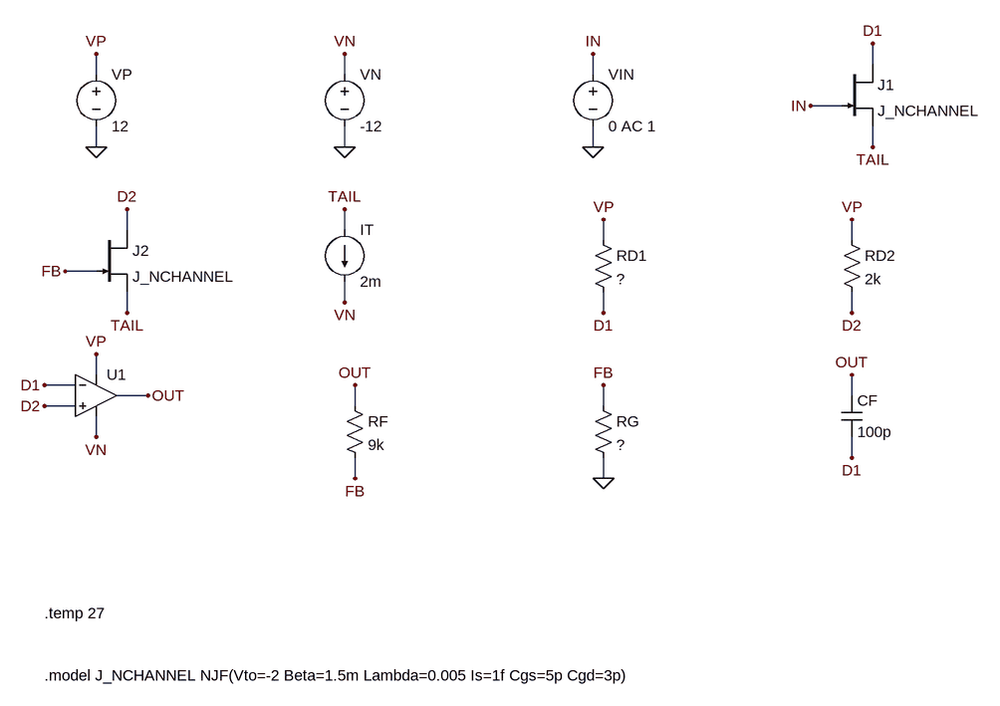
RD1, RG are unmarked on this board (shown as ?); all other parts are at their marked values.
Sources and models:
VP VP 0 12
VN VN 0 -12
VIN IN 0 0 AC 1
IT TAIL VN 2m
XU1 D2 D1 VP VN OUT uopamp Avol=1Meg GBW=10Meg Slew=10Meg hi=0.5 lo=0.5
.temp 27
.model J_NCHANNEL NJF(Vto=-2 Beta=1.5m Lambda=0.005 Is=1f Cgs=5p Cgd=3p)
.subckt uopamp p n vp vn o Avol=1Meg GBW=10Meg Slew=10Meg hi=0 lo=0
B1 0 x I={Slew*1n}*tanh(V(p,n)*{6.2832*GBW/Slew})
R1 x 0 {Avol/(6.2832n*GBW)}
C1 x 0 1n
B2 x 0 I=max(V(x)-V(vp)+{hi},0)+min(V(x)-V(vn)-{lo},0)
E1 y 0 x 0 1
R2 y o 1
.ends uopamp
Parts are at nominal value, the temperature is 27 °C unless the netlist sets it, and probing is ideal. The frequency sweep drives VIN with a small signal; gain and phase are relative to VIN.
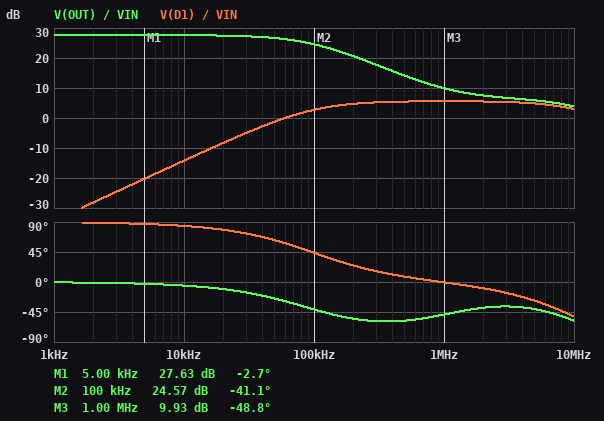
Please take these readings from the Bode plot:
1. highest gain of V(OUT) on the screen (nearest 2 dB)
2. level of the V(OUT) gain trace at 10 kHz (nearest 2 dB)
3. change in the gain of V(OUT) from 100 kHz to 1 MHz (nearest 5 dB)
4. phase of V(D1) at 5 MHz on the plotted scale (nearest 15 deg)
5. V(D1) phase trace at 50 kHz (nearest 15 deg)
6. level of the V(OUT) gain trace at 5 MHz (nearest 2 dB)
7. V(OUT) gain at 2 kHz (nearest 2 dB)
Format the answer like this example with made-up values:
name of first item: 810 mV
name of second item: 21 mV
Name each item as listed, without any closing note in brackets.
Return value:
highest gain of V(OUT) on the screen: 28 dB
level of the V(OUT) gain trace at 10 kHz: 28 dB
change in the gain of V(OUT) from 100 kHz to 1 MHz: -15 dB
phase of V(D1) at 5 MHz on the plotted scale: -30 deg
V(D1) phase trace at 50 kHz: 60 deg
level of the V(OUT) gain trace at 5 MHz: 6 dB
V(OUT) gain at 2 kHz: 28 dB
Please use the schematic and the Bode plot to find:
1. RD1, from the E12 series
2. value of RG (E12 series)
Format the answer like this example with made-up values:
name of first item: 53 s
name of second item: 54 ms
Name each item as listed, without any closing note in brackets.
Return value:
RD1, from the E12 series: 4.7 kΩ
value of RG: 390 Ω
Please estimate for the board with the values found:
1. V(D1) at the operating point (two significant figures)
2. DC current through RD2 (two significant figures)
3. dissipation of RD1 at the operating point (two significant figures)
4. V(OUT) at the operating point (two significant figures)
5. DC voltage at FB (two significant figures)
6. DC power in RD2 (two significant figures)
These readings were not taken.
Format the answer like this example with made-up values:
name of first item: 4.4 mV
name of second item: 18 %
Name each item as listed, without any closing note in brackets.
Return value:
V(D1) at the operating point: 9.2 V
DC current through RD2: 1.4 mA
dissipation of RD1 at the operating point: 1.7 mW
V(OUT) at the operating point: 7.9 V
DC voltage at FB: 330 mV
DC power in RD2: 3.9 mW
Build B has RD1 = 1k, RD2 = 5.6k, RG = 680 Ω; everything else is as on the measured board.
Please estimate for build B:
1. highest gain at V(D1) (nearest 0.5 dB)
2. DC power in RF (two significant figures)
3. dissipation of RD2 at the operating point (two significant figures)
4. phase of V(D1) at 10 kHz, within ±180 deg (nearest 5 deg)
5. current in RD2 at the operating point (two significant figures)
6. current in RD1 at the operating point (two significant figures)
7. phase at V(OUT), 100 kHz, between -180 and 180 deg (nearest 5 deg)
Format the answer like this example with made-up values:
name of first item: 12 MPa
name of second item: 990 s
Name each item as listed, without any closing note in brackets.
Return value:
highest gain at V(D1): 11.0 dB
DC power in RF: 7.0 mW
dissipation of RD2 at the operating point: 510 µW
phase of V(D1) at 10 kHz, within ±180 deg: 90 deg
current in RD2 at the operating point: 300 µA
current in RD1 at the operating point: 1.7 mA
phase at V(OUT), 100 kHz, between -180 and 180 deg: -10 deg
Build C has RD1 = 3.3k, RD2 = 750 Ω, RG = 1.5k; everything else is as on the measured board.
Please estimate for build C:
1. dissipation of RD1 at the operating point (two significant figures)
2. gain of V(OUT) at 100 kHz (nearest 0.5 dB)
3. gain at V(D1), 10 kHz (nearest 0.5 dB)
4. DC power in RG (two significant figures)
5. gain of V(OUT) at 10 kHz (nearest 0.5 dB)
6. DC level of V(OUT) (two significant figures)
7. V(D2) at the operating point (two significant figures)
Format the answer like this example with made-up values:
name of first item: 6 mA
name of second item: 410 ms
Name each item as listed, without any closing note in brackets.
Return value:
dissipation of RD1 at the operating point: 450 µW
gain of V(OUT) at 100 kHz: 16.5 dB
gain at V(D1), 10 kHz: -33.5 dB
DC power in RG: 190 µW
gain of V(OUT) at 10 kHz: 17.0 dB
DC level of V(OUT): 3.7 V
V(D2) at the operating point: 11 V
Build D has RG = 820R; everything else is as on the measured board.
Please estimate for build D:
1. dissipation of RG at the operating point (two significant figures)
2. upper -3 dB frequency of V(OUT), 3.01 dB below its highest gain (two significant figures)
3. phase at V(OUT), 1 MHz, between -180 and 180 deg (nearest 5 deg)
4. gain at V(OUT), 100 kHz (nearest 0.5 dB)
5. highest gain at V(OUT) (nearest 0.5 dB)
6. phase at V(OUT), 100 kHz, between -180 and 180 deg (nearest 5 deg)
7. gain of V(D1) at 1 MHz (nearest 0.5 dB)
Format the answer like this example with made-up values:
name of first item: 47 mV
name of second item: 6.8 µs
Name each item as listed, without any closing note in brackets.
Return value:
dissipation of RG at the operating point: 130 µW
upper -3 dB frequency of V(OUT), 3.01 dB below its highest gain: 190 kHz
phase at V(OUT), 1 MHz, between -180 and 180 deg: -45 deg
gain at V(OUT), 100 kHz: 20.5 dB
highest gain at V(OUT): 21.5 dB
phase at V(OUT), 100 kHz, between -180 and 180 deg: -25 deg
gain of V(D1) at 1 MHz: 5.0 dB
